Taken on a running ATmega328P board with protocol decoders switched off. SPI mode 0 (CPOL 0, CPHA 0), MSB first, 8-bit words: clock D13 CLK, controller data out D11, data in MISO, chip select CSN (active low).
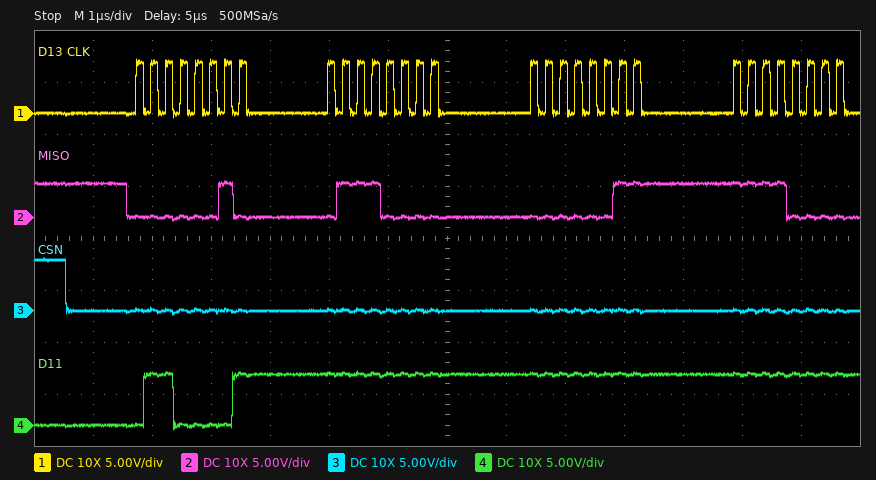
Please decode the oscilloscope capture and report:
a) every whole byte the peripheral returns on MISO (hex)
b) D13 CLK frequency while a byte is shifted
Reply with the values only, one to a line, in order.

02 70 03 F0
4 MHz
